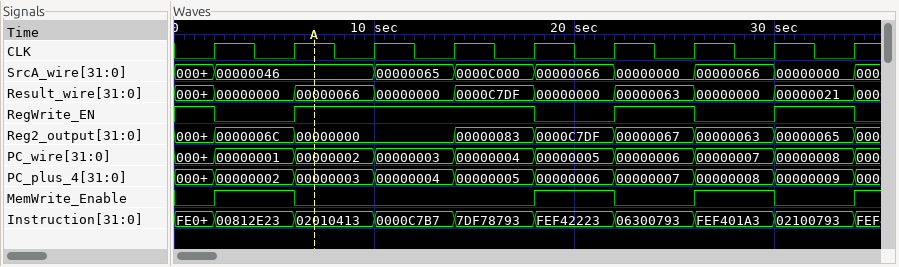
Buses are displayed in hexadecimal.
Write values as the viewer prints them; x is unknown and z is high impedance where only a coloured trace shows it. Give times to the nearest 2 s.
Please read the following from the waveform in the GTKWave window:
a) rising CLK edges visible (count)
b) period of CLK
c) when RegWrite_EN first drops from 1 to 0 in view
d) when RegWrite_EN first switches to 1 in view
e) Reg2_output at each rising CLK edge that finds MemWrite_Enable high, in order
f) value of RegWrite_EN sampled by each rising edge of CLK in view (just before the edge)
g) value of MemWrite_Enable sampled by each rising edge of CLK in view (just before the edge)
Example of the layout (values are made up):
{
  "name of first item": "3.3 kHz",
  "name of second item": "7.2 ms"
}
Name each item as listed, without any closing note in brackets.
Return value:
{
  "rising CLK edges visible": "9",
  "period of CLK": "4 s",
  "when RegWrite_EN first drops from 1 to 0 in view": "2 s",
  "when RegWrite_EN first switches to 1 in view": "6 s",
  "Reg2_output at each rising CLK edge that finds MemWrite_Enable high, in order": "0000006C, 0000C7DF, 00000063",
  "value of RegWrite_EN sampled by each rising edge of CLK in view": "1 0 1 1 1 0 1 0 1",
  "value of MemWrite_Enable sampled by each rising edge of CLK in view": "0 1 0 0 0 1 0 1 0"
}
